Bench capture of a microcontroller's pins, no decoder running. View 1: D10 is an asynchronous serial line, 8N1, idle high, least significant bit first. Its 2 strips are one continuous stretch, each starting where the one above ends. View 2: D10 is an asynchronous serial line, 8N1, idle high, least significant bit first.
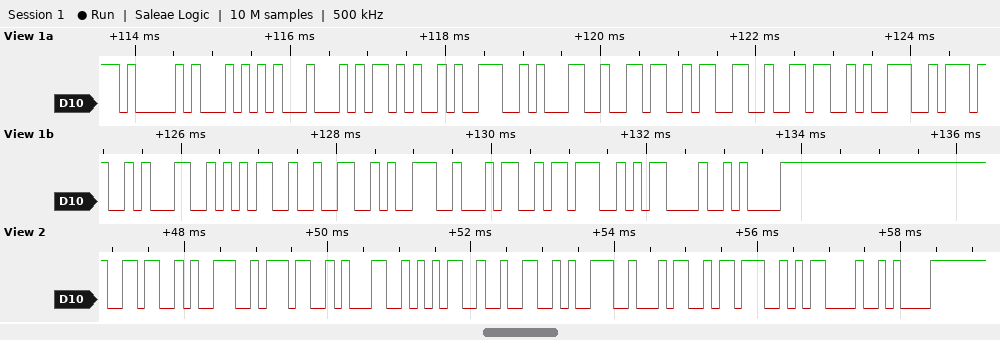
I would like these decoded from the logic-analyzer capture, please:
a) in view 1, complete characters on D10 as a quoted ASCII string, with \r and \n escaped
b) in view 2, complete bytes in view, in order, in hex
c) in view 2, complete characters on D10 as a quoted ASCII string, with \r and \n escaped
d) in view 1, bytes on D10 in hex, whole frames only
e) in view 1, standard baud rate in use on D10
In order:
"ATD+916369715294;\r\n"
36 39 37 31 35 32 39 34 3B 0D 0A
"69715294;\r\n"
41 54 44 2B 39 31 36 33 36 39 37 31 35 32 39 34 3B 0D 0A
9600 baud
